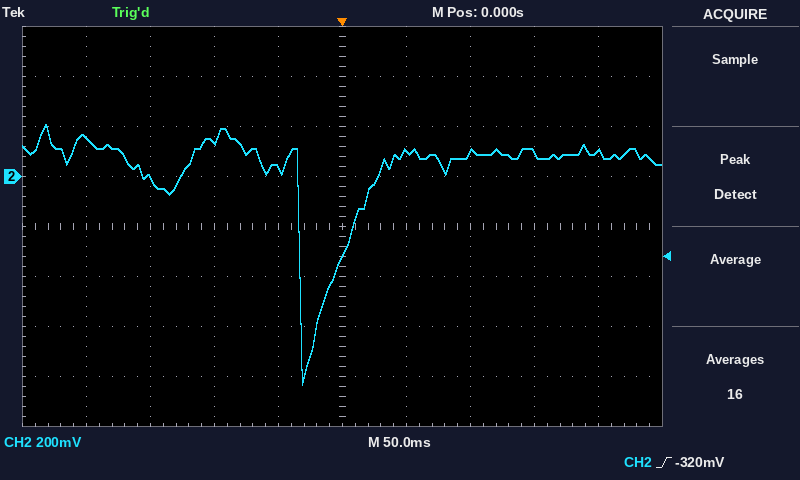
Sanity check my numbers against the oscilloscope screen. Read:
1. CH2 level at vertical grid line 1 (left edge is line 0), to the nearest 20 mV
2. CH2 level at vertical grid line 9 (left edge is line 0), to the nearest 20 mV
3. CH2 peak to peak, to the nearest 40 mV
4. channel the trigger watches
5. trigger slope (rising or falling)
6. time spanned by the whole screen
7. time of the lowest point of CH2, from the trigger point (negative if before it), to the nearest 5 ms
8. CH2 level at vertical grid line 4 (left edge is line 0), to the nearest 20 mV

160 mV
100 mV
1.04 V
CH2
rising
500 ms
-30 ms
40 mV
